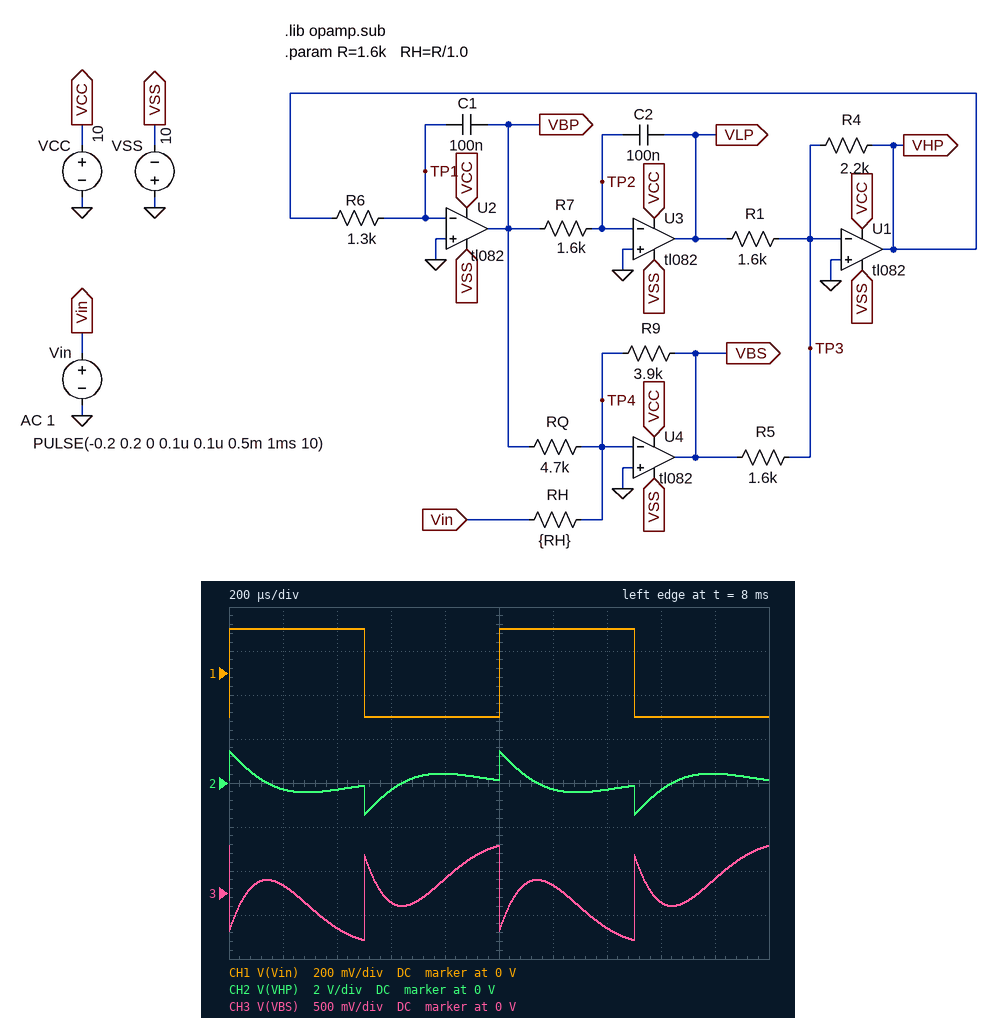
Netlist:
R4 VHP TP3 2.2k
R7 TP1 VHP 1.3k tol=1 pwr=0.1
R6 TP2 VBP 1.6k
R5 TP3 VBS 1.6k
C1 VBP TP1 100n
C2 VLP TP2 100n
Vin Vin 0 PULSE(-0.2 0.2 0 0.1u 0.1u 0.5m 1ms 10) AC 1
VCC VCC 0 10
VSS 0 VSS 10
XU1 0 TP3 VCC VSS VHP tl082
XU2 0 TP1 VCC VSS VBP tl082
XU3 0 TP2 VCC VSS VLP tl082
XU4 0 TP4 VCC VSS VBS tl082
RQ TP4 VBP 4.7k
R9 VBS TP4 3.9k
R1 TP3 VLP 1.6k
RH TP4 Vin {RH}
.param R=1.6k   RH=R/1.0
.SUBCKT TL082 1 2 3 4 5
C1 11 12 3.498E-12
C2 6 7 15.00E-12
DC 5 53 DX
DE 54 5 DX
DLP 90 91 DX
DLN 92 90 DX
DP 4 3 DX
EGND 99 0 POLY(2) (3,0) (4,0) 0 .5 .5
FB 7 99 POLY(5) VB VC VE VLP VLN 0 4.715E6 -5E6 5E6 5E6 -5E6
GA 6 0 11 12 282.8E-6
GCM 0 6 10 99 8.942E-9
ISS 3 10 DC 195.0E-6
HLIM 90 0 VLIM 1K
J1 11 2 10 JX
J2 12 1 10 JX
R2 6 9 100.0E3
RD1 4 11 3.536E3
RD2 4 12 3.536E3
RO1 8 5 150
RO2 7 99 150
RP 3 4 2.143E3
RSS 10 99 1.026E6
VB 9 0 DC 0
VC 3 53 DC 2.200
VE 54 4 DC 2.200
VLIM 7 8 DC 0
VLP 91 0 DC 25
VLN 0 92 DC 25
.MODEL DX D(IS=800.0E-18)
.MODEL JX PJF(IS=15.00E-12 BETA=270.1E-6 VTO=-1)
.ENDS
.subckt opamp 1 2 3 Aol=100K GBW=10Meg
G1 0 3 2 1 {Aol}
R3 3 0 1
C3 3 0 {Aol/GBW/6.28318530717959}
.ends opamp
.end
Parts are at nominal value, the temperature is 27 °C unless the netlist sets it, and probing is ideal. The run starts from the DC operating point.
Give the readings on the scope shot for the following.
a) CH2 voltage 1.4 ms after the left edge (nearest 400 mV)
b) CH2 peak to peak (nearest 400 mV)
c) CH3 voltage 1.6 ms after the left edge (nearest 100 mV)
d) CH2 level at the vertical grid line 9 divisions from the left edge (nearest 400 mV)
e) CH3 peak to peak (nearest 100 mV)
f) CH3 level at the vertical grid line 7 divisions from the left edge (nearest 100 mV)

-400 mV
2.8 V
-100 mV
400 mV
1.1 V
-400 mV
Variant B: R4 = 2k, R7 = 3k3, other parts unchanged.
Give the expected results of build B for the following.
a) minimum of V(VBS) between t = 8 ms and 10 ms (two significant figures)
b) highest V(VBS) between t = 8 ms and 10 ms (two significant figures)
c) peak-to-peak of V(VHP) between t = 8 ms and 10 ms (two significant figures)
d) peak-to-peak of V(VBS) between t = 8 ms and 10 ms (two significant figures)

-860 mV
860 mV
3.3 V
1.7 V
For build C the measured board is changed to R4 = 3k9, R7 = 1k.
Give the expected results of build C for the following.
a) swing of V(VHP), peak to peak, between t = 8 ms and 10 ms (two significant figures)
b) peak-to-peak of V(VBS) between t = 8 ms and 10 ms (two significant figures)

4.7 V
990 mV
